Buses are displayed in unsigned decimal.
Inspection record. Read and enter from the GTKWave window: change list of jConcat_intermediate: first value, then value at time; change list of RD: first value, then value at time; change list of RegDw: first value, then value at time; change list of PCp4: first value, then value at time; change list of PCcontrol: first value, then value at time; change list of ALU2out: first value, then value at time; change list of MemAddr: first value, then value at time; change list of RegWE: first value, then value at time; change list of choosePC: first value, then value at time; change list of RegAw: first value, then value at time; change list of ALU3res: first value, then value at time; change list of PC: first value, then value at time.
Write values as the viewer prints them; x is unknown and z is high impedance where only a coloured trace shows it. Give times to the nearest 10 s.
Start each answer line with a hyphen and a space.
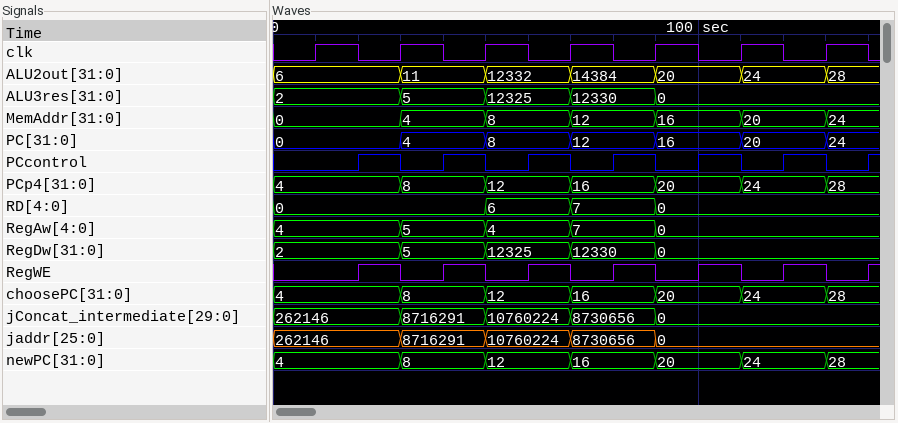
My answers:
- 262146, 8716291 at 30 s, 10760224 at 50 s, 8730656 at 70 s, 0 at 90 s
- 0, 6 at 50 s, 7 at 70 s, 0 at 90 s
- 2, 5 at 30 s, 12325 at 50 s, 12330 at 70 s, 0 at 90 s
- 4, 8 at 30 s, 12 at 50 s, 16 at 70 s, 20 at 90 s, 24 at 110 s, 28 at 130 s
- 0, 1 at 20 s, 0 at 30 s, 1 at 40 s, 0 at 50 s, 1 at 60 s, 0 at 70 s, 1 at 80 s, 0 at 90 s, 1 at 100 s, 0 at 110 s, 1 at 120 s, 0 at 130 s, 1 at 140 s
- 6, 11 at 30 s, 12332 at 50 s, 14384 at 70 s, 20 at 90 s, 24 at 110 s, 28 at 130 s
- 0, 4 at 30 s, 8 at 50 s, 12 at 70 s, 16 at 90 s, 20 at 110 s, 24 at 130 s
- 0, 1 at 20 s, 0 at 30 s, 1 at 40 s, 0 at 50 s, 1 at 60 s, 0 at 70 s, 1 at 80 s, 0 at 90 s, 1 at 100 s, 0 at 110 s, 1 at 120 s, 0 at 130 s, 1 at 140 s
- 4, 8 at 30 s, 12 at 50 s, 16 at 70 s, 20 at 90 s, 24 at 110 s, 28 at 130 s
- 4, 5 at 30 s, 4 at 50 s, 7 at 70 s, 0 at 90 s
- 2, 5 at 30 s, 12325 at 50 s, 12330 at 70 s, 0 at 90 s
- 0, 4 at 30 s, 8 at 50 s, 12 at 70 s, 16 at 90 s, 20 at 110 s, 24 at 130 s
